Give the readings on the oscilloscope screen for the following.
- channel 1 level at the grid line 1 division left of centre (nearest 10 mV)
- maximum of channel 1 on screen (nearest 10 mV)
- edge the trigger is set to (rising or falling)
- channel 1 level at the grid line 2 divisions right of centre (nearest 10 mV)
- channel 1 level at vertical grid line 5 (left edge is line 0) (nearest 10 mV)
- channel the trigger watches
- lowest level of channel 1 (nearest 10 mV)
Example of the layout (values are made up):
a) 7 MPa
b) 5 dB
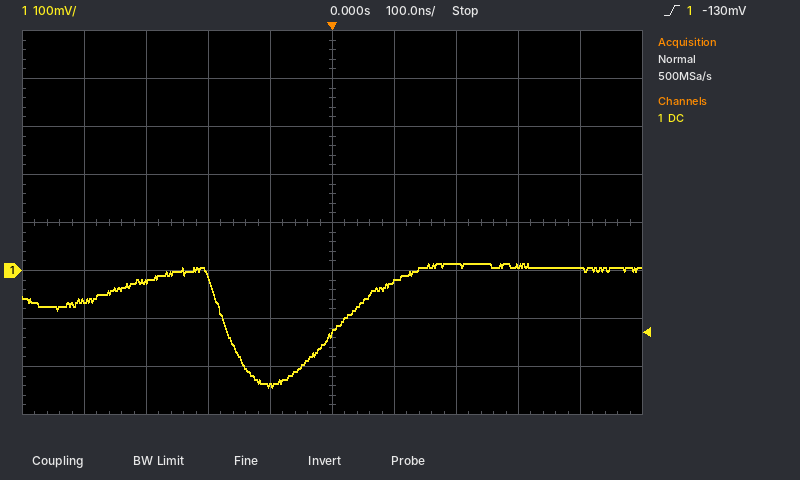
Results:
a) -240 mV
b) 10 mV
c) rising
d) 10 mV
e) -130 mV
f) channel 1
g) -240 mV
